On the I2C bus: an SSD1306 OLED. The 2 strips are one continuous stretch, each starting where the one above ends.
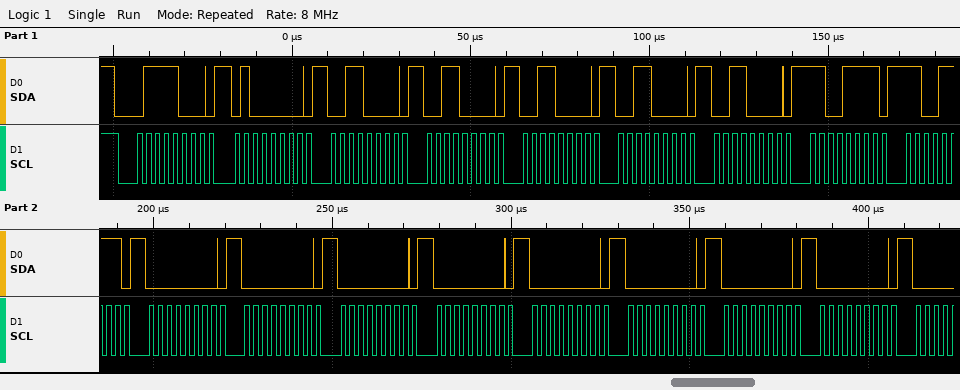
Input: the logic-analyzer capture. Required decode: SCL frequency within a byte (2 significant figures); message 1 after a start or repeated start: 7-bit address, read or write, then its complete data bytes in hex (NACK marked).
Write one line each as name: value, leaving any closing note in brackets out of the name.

SCL frequency within a byte: 400 kHz
message 1 after a start or repeated start: 7-bit address, read or write, then its complete data bytes in hex: 0x3C write: 40 30 30 30 30 30 CF CF 00 00 00 00 00 00 00 00
